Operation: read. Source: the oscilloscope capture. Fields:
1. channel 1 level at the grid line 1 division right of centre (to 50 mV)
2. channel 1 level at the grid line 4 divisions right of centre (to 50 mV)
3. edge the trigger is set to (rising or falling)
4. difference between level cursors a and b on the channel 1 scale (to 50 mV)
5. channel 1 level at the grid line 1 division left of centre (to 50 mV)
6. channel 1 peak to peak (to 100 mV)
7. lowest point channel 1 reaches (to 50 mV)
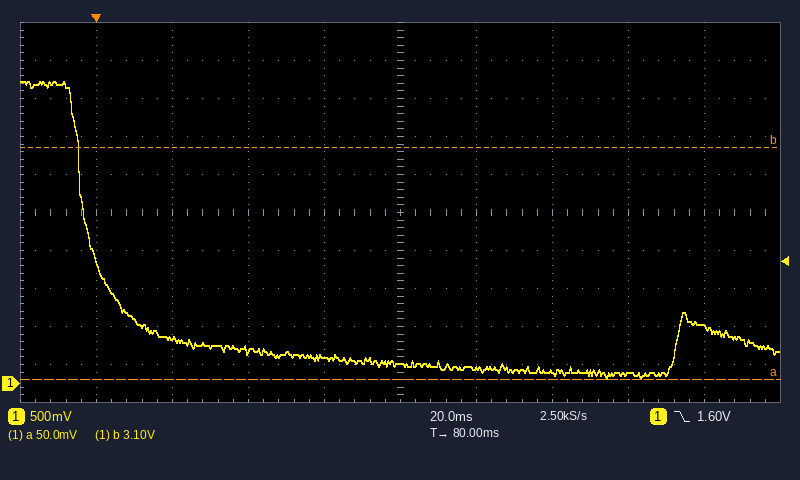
200 mV
750 mV
falling
3.05 V
350 mV
3.90 V
50 mV
